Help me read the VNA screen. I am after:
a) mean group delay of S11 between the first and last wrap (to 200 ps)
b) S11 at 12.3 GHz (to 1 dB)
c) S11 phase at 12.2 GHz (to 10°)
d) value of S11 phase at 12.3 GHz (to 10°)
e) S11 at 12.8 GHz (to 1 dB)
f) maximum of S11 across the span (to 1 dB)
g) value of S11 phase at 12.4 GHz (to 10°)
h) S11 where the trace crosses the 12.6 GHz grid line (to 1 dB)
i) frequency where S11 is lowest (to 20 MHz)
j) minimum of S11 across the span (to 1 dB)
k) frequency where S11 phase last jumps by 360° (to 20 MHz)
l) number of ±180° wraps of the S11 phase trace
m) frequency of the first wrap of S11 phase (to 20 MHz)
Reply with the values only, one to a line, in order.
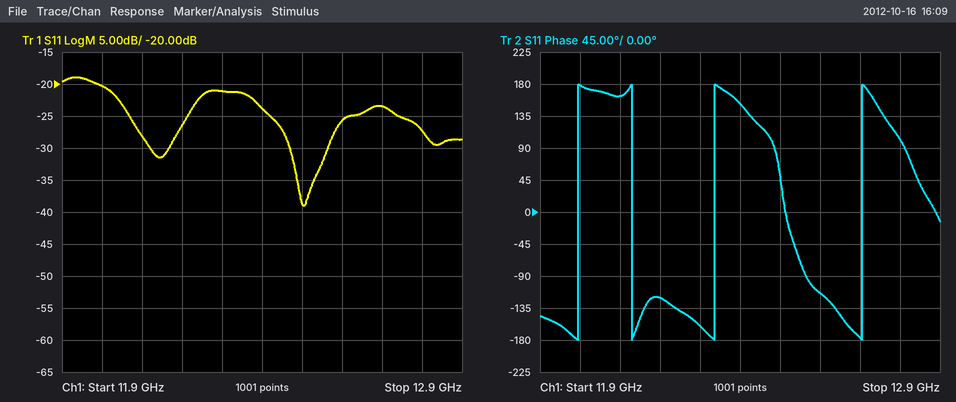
4.2 ns
-21 dB
-120°
-160°
-27 dB
-19 dB
150°
-26 dB
12.50 GHz
-39 dB
12.70 GHz
4
12.00 GHz
